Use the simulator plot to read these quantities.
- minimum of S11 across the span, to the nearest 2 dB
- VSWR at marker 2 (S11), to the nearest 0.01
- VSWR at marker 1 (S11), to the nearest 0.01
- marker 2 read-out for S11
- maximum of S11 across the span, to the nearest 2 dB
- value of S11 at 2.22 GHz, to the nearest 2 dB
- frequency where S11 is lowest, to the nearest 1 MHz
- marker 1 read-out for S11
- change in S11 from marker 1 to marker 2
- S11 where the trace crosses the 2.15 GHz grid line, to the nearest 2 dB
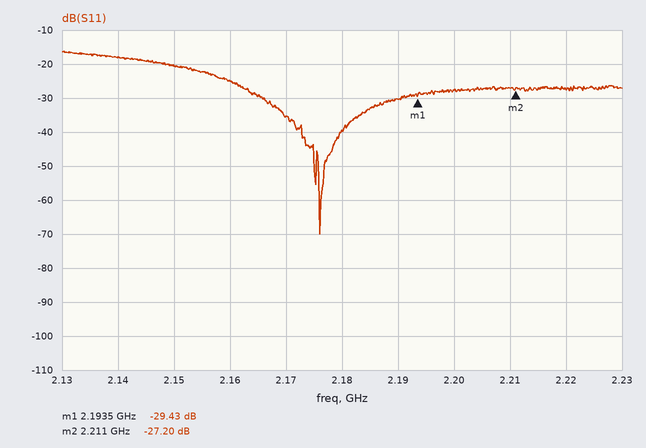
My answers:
-70 dB
1.09
1.07
-27.20 dB
-16 dB
-28 dB
2.176 GHz
-29.43 dB
2.23 dB
-20 dB
